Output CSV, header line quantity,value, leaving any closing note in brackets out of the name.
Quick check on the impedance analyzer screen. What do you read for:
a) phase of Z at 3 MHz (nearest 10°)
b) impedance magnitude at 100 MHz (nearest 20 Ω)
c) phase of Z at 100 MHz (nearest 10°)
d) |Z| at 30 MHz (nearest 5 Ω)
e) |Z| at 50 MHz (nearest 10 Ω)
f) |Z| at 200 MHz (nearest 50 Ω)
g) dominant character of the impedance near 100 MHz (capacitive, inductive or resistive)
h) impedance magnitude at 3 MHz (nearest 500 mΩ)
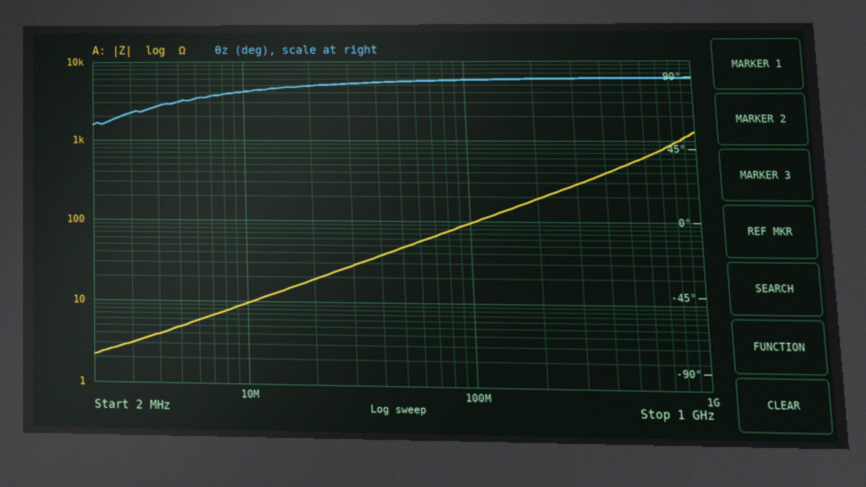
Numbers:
quantity,value
phase of Z at 3 MHz,70°
impedance magnitude at 100 MHz,100 Ω
phase of Z at 100 MHz,90°
|Z| at 30 MHz,30 Ω
|Z| at 50 MHz,50 Ω
|Z| at 200 MHz,200 Ω
dominant character of the impedance near 100 MHz,inductive
impedance magnitude at 3 MHz,3.0 Ω
